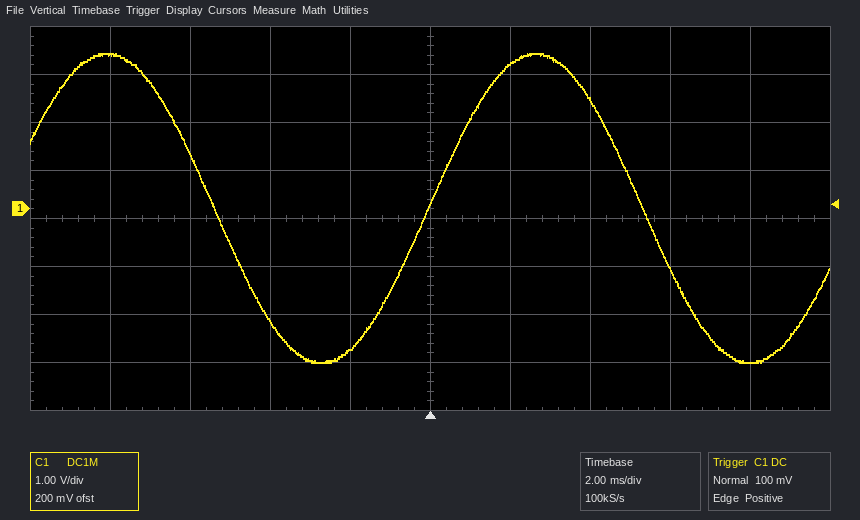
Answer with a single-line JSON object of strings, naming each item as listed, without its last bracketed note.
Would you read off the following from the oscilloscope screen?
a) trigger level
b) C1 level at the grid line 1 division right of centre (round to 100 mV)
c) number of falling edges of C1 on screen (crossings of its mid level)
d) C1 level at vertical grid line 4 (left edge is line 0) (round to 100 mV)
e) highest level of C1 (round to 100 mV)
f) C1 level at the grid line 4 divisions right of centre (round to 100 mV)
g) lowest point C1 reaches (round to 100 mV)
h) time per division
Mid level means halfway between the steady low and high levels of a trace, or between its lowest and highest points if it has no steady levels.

{"trigger level": "100 mV", "C1 level at the grid line 1 division right of centre": "3.0 V", "number of falling edges of C1 on screen": "2", "C1 level at vertical grid line 4 (left edge is line 0)": "-2.9 V", "highest level of C1": "3.2 V", "C1 level at the grid line 4 divisions right of centre": "-3.2 V", "lowest point C1 reaches": "-3.2 V", "time per division": "2 ms"}
